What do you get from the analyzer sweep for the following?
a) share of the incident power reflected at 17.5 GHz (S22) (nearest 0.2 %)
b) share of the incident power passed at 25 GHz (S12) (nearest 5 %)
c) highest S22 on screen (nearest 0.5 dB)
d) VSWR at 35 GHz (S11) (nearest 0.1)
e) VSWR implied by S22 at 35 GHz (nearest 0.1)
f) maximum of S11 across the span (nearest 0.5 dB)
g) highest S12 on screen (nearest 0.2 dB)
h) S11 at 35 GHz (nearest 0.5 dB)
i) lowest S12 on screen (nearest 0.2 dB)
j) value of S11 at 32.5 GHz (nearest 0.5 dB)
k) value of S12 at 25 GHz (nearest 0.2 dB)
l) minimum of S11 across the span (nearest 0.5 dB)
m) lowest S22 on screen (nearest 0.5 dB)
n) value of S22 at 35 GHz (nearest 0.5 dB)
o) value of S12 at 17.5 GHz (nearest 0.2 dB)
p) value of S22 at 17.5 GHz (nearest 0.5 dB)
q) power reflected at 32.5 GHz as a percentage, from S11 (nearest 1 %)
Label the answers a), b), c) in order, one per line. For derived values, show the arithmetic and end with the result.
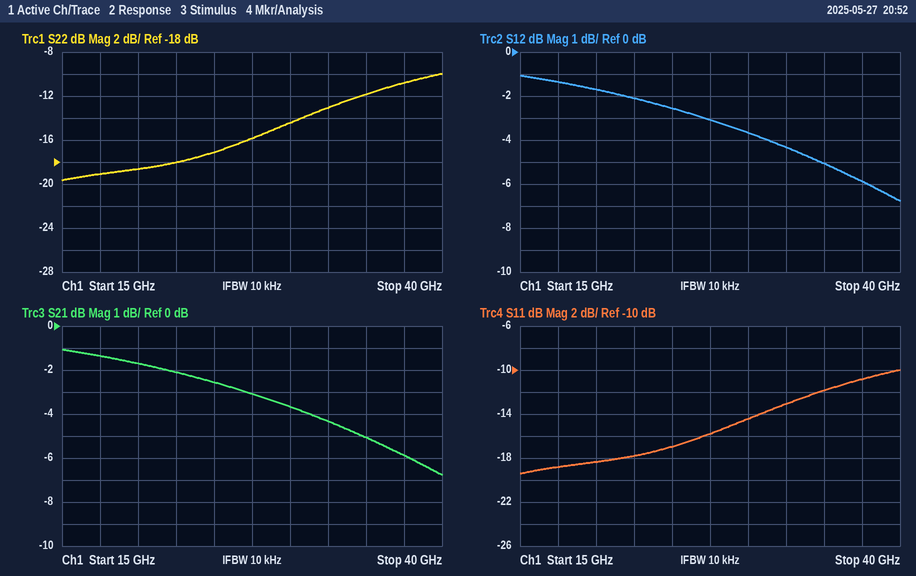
a) 10^(-19/10) ≈ 1.26 %, so 1.2 % to the nearest 0.2 %
b) 10^(-2.6/10) ≈ 55 %
c) -10.0 dB
d) |Γ| = 10^(-12/20) = 0.2512; VSWR = (1 + 0.2512)/(1 − 0.2512) ≈ 1.7
e) |Γ| = 10^(-12/20) = 0.2512; VSWR = (1 + 0.2512)/(1 − 0.2512) ≈ 1.7
f) -10.0 dB
g) -1.0 dB
h) -12.0 dB
i) -6.8 dB
j) -13.0 dB
k) -2.6 dB
l) -19.5 dB
m) -19.5 dB
n) -12.0 dB
o) -1.4 dB
p) -19.0 dB
q) 10^(-13/10) ≈ 5 %
